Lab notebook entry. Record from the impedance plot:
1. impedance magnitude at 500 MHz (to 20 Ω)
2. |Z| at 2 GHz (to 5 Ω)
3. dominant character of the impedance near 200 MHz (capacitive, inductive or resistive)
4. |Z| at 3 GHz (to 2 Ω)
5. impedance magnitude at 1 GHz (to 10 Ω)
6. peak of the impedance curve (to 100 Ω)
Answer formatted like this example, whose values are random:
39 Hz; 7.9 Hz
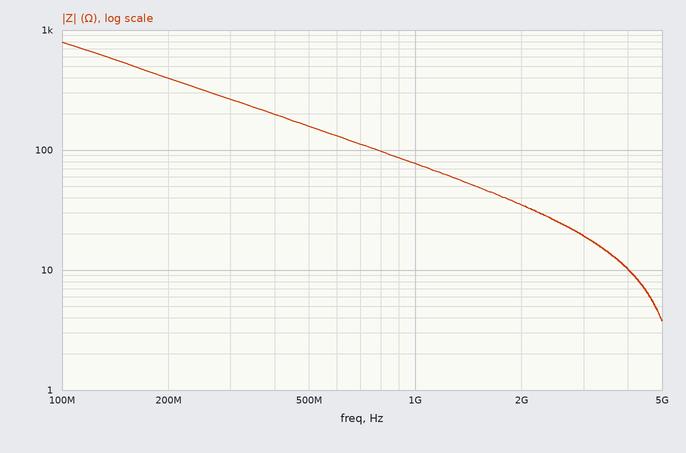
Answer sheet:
160 Ω; 35 Ω; capacitive; 20 Ω; 80 Ω; 800 Ω
